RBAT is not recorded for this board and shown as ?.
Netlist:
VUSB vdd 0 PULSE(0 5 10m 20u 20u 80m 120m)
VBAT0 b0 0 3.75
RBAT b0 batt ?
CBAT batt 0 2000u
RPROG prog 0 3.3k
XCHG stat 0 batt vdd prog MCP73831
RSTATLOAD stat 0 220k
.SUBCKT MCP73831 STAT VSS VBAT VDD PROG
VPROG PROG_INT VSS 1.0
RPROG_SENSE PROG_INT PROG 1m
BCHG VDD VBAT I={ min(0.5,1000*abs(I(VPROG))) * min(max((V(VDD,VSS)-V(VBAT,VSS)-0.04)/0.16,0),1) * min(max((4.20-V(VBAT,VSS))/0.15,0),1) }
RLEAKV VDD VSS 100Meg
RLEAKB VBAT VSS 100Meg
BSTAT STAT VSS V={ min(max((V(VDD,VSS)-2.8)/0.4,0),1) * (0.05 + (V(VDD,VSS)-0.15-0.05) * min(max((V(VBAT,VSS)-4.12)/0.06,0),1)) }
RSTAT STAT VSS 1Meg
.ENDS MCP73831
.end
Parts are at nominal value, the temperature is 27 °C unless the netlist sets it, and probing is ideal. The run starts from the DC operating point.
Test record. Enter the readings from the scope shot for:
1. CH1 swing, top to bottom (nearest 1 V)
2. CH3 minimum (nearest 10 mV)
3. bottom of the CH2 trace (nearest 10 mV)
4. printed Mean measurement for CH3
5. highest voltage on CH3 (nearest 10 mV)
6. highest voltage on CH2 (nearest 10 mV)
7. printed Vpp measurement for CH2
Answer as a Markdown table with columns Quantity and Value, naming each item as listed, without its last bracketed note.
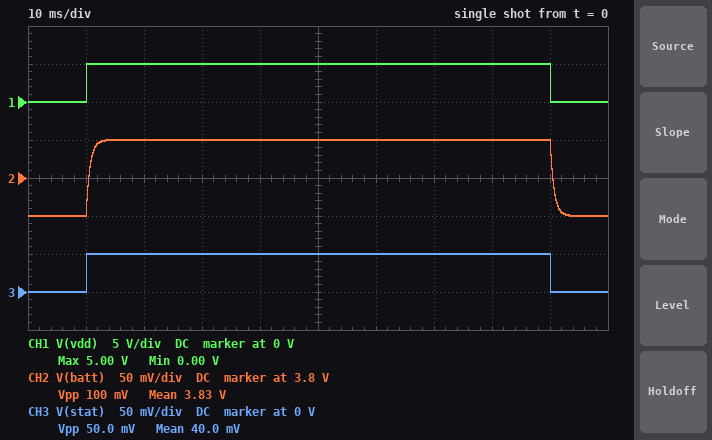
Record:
| Quantity | Value |
|---|---|
| CH1 swing, top to bottom | 5 V |
| CH3 minimum | 0 V |
| bottom of the CH2 trace | 3.75 V |
| printed Mean measurement for CH3 | 40.0 mV |
| highest voltage on CH3 | 50 mV |
| highest voltage on CH2 | 3.85 V |
| printed Vpp measurement for CH2 | 100 mV |
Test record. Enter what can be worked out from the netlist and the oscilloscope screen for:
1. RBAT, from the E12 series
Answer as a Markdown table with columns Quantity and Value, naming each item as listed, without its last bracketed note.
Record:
| Quantity | Value |
|---|---|
| RBAT, from the E12 series | 0.33 Ω |
